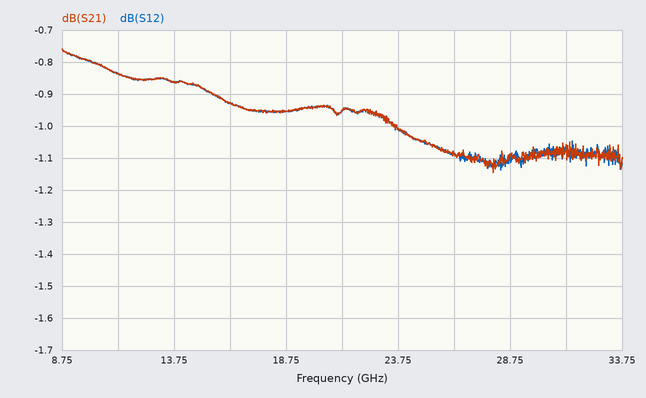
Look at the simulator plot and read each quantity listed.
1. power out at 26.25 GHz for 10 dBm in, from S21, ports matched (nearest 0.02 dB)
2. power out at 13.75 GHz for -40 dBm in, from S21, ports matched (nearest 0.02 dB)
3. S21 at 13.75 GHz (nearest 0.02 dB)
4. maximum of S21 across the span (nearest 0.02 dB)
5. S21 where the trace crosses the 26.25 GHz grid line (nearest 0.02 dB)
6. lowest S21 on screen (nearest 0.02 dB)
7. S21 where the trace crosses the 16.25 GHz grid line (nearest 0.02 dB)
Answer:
8.92 dBm
-40.86 dBm
-0.86 dB
-0.76 dB
-1.08 dB
-1.14 dB
-0.92 dB
